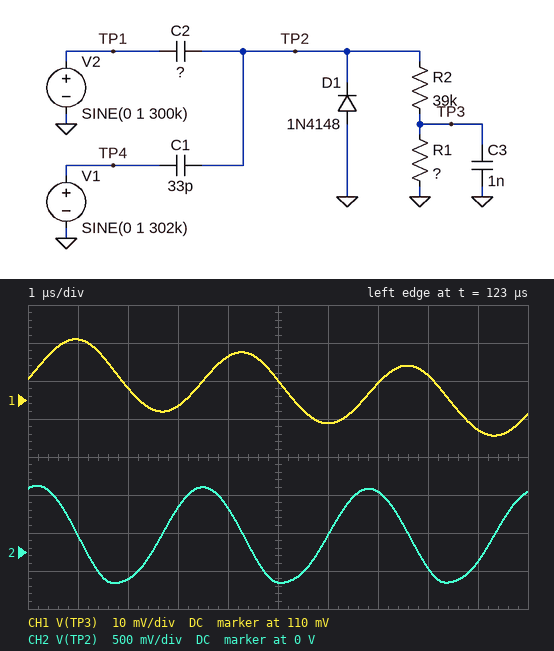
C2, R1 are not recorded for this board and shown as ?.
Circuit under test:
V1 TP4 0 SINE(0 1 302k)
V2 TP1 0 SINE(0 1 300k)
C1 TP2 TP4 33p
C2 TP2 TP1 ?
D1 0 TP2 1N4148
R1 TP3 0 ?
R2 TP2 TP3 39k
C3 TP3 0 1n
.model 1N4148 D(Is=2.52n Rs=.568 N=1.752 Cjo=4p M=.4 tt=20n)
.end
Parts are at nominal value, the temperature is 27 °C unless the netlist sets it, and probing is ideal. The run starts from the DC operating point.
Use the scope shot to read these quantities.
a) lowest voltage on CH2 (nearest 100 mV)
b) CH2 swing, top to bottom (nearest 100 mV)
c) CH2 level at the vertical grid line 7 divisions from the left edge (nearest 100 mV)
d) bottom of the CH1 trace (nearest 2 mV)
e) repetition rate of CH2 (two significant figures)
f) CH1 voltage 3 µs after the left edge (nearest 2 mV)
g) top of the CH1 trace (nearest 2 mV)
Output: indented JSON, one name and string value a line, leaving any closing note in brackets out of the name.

{
  "lowest voltage on CH2": "-400 mV",
  "CH2 swing, top to bottom": "1.3 V",
  "CH2 level at the vertical grid line 7 divisions from the left edge": "800 mV",
  "bottom of the CH1 trace": "100 mV",
  "repetition rate of CH2": "300 kHz",
  "CH1 voltage 3 µs after the left edge": "108 mV",
  "top of the CH1 trace": "126 mV"
}
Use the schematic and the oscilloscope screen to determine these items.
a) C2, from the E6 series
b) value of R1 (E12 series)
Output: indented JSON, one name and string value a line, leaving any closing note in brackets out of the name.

{
  "C2, from the E6 series": "22 pF",
  "value of R1": "33 kΩ"
}
